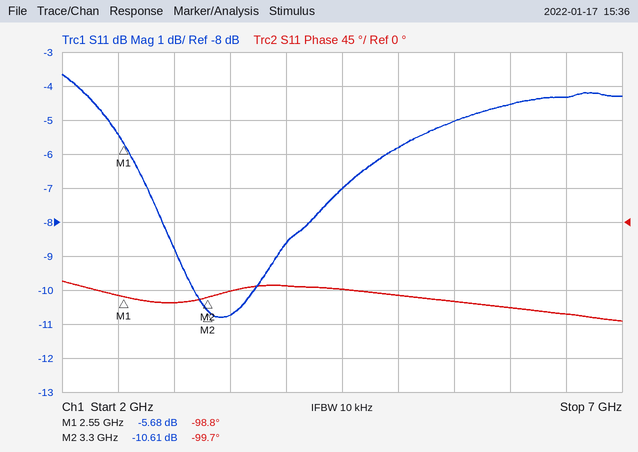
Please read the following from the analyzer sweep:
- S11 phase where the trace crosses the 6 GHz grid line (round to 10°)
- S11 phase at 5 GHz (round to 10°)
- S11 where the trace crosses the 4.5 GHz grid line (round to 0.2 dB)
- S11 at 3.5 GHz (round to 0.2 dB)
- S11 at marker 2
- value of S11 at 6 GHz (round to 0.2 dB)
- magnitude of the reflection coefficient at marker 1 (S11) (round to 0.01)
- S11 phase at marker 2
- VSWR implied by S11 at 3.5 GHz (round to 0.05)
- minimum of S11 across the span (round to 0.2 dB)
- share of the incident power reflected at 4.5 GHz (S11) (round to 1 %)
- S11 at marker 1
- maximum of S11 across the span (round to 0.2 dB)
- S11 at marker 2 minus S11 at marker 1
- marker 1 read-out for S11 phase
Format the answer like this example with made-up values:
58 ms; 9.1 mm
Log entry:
-110°; -100°; -7.0 dB; -10.8 dB; -10.61 dB; -4.6 dB; 0.52; -99.7°; 1.80; -10.8 dB; 20 %; -5.68 dB; -3.6 dB; -4.93 dB; -98.8°
